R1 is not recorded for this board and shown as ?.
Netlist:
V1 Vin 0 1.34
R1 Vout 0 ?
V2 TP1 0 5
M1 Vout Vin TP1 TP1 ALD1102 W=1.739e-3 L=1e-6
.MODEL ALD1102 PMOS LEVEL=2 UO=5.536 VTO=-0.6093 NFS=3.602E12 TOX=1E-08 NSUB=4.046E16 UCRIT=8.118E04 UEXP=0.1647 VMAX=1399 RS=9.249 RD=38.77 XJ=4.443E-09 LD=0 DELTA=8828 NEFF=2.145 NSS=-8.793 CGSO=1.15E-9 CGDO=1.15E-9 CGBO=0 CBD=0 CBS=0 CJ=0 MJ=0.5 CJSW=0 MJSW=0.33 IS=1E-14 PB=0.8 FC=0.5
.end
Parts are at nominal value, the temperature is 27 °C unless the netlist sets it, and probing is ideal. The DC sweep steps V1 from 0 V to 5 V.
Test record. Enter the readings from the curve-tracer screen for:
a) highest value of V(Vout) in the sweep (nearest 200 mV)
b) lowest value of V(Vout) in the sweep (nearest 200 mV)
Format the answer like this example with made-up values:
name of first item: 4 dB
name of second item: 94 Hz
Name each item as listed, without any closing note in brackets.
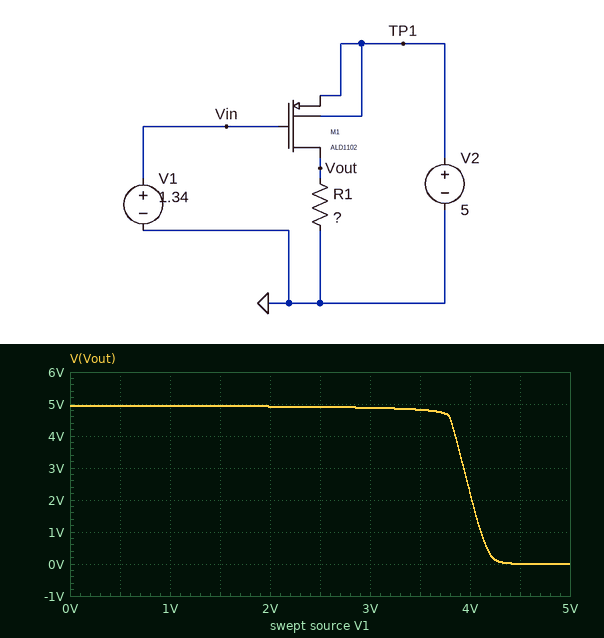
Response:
highest value of V(Vout) in the sweep: 5.0 V
lowest value of V(Vout) in the sweep: 0 V
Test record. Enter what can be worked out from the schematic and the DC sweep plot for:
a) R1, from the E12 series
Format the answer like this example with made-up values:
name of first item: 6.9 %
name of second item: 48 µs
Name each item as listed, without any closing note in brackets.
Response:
R1, from the E12 series: 15 kΩ
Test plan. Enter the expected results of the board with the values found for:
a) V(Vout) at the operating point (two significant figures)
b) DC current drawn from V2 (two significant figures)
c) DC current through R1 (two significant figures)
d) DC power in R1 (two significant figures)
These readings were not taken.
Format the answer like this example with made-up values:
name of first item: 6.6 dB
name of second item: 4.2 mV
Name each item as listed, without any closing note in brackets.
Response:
V(Vout) at the operating point: 4.9 V
DC current drawn from V2: 330 µA
DC current through R1: 330 µA
DC power in R1: 1.6 mW
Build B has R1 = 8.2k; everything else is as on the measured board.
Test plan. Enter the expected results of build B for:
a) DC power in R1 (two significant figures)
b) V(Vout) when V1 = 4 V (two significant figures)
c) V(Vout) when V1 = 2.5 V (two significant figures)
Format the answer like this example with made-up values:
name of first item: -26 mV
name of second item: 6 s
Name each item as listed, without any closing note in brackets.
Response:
DC power in R1: 2.9 mW
V(Vout) when V1 = 4 V: 1.3 V
V(Vout) when V1 = 2.5 V: 4.8 V
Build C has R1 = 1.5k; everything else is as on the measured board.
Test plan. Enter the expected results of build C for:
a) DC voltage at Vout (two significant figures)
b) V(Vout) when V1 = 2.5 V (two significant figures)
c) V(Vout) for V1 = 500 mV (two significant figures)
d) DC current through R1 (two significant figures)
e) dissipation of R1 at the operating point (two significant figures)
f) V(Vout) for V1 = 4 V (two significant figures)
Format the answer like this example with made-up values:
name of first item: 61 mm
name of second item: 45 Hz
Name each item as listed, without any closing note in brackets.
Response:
DC voltage at Vout: 4.4 V
V(Vout) when V1 = 2.5 V: 4.0 V
V(Vout) for V1 = 500 mV: 4.5 V
DC current through R1: 2.9 mA
dissipation of R1 at the operating point: 13 mW
V(Vout) for V1 = 4 V: 240 mV
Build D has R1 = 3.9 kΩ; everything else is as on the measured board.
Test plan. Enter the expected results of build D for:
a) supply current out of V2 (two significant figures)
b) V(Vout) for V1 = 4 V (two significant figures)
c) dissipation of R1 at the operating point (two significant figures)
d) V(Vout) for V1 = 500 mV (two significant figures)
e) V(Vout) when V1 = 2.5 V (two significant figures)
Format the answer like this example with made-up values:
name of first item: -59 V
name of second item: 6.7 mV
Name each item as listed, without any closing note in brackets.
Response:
supply current out of V2: 1.2 mA
V(Vout) for V1 = 4 V: 620 mV
dissipation of R1 at the operating point: 5.8 mW
V(Vout) for V1 = 500 mV: 4.8 V
V(Vout) when V1 = 2.5 V: 4.6 V
